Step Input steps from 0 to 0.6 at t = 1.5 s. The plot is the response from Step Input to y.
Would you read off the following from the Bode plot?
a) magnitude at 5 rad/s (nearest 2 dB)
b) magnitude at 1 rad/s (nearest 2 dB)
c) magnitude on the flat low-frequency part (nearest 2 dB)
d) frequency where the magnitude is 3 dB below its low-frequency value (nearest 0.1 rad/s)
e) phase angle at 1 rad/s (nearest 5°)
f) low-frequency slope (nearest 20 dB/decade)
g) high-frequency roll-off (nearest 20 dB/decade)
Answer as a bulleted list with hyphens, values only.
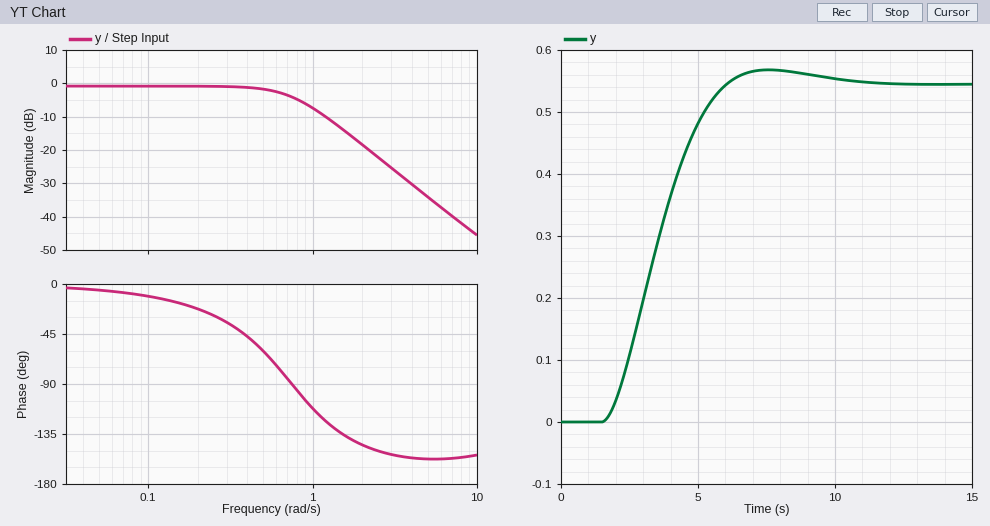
- -34 dB
- -8 dB
- 0 dB
- 0.7 rad/s
- -110°
- 0 dB/decade
- -40 dB/decade
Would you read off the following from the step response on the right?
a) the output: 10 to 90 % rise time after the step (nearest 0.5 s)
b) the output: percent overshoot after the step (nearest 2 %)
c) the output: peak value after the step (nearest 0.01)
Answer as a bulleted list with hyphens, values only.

- 3.0 s
- 4 %
- 0.57
